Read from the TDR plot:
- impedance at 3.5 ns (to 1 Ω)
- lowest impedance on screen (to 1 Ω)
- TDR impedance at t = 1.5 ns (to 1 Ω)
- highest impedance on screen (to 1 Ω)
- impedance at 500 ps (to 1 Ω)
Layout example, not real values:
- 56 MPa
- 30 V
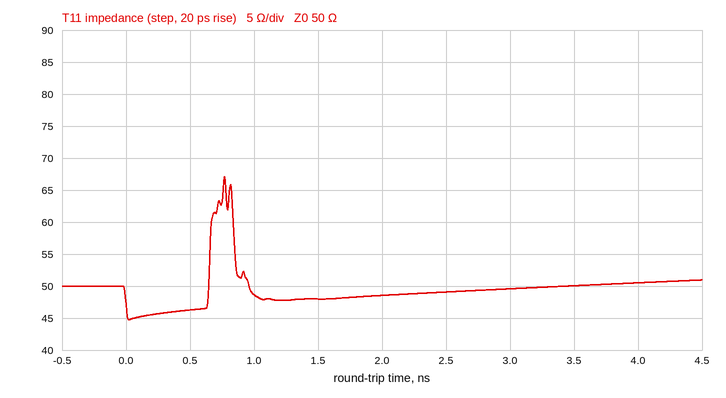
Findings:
- 50 Ω
- 45 Ω
- 48 Ω
- 67 Ω
- 46 Ω
